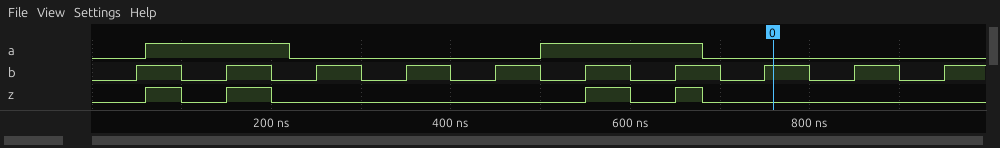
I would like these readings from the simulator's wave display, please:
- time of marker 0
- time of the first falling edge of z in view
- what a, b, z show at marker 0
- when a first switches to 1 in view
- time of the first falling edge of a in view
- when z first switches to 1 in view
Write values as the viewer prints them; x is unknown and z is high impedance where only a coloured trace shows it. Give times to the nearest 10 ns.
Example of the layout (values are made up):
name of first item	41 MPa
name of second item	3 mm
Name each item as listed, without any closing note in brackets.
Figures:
time of marker 0	760 ns
time of the first falling edge of z in view	100 ns
what a, b, z show at marker 0	a=0, b=1, z=0
when a first switches to 1 in view	60 ns
time of the first falling edge of a in view	220 ns
when z first switches to 1 in view	60 ns
